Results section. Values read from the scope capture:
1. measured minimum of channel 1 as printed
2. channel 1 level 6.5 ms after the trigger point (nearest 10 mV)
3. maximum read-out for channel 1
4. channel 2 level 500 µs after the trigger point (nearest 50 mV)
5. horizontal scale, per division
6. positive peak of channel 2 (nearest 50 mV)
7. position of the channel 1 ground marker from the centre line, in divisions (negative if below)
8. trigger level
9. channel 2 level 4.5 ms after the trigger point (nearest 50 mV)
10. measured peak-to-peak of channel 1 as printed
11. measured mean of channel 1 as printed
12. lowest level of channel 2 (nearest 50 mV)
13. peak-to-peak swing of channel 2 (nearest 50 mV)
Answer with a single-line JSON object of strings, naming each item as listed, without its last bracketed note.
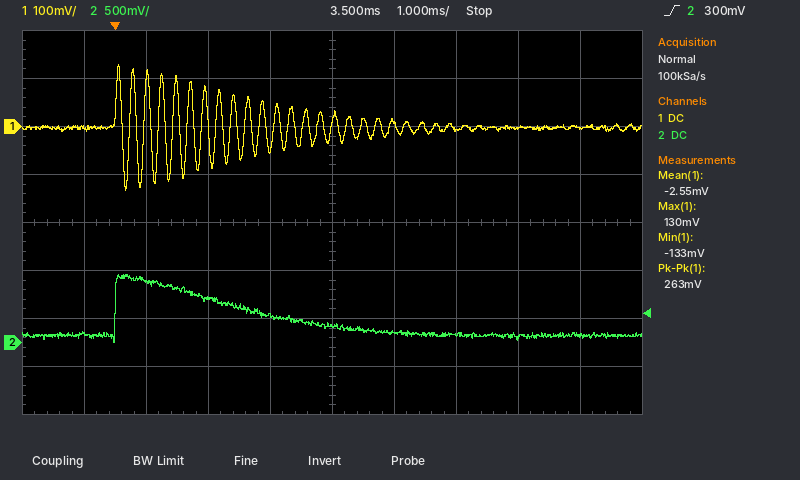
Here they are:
{"measured minimum of channel 1 as printed": "-133 mV", "channel 1 level 6.5 ms after the trigger point": "0 mV", "maximum read-out for channel 1": "130 mV", "channel 2 level 500 µs after the trigger point": "650 mV", "horizontal scale, per division": "1 ms", "positive peak of channel 2": "700 mV", "position of the channel 1 ground marker from the centre line, in divisions": "+2.0 div", "trigger level": "300 mV", "channel 2 level 4.5 ms after the trigger point": "100 mV", "measured peak-to-peak of channel 1 as printed": "263 mV", "measured mean of channel 1 as printed": "-2.55 mV", "lowest level of channel 2": "0 mV", "peak-to-peak swing of channel 2": "700 mV"}
